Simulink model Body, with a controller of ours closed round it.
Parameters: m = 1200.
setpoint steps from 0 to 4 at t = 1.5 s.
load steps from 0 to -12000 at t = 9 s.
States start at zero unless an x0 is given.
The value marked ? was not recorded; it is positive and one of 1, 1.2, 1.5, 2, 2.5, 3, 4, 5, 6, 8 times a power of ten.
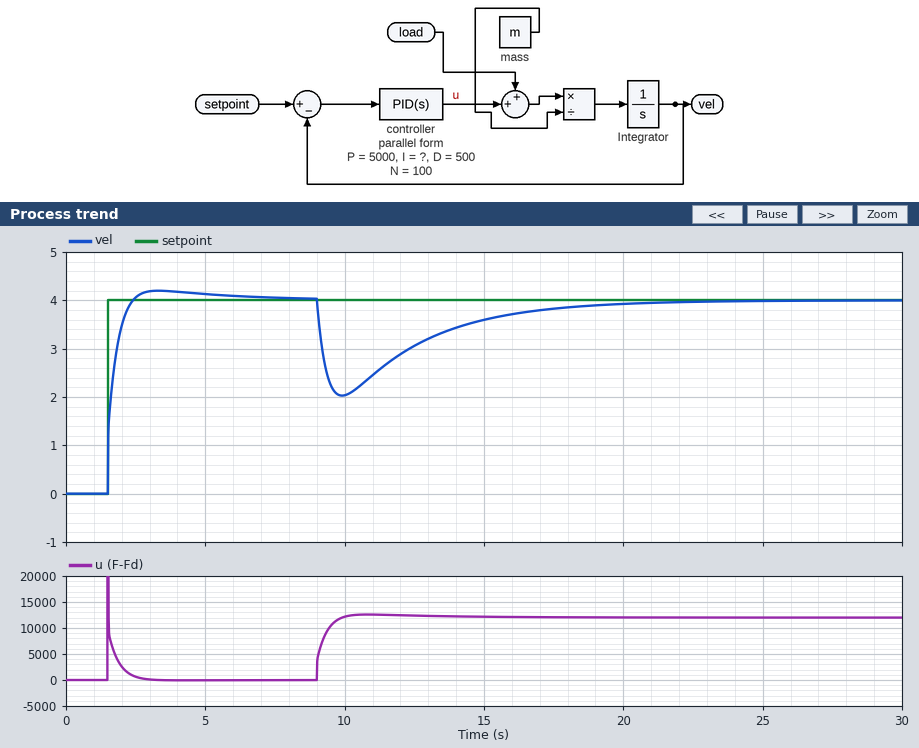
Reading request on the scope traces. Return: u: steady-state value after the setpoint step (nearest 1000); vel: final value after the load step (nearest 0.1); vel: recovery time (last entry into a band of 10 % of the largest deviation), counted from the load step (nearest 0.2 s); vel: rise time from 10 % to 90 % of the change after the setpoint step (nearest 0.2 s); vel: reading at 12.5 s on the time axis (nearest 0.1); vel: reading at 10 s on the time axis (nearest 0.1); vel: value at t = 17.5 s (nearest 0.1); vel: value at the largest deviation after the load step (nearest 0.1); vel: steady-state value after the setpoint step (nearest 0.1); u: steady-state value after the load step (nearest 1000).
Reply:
0
4.0
8.0 s
0.6 s
3.1
2.0
3.8
2.0
4.0
12000
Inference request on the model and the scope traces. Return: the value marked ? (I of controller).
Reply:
1500
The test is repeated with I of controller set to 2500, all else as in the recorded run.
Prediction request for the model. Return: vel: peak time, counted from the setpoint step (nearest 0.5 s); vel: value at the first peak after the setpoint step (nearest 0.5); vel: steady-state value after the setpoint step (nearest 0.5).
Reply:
1.5 s
4.5
4.0
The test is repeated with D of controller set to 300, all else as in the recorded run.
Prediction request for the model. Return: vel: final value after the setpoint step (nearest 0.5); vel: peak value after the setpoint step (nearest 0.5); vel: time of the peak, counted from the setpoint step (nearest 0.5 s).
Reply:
4.0
4.0
1.5 s
